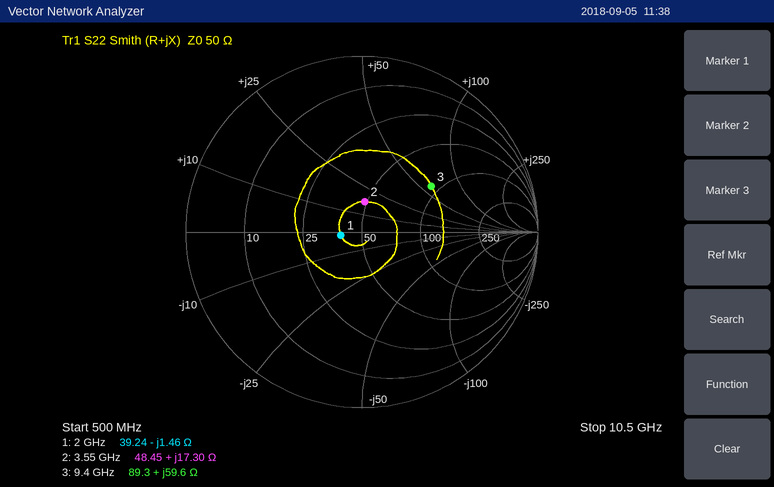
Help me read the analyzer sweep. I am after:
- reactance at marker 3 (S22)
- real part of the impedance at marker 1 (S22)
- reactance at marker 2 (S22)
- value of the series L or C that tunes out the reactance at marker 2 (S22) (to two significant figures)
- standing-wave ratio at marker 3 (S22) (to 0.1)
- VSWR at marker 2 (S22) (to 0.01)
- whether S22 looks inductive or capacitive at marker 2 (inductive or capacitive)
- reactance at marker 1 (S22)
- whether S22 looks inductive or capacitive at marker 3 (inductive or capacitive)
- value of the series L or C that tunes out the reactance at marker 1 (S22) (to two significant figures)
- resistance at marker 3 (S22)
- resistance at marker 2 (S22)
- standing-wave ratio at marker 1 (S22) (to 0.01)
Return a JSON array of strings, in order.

["+59.6 Ω", "39.24 Ω", "+17.30 Ω", "2.6 pF", "2.8", "1.42", "inductive", "-1.46 Ω", "inductive", "120 pH", "89.3 Ω", "48.45 Ω", "1.28"]
